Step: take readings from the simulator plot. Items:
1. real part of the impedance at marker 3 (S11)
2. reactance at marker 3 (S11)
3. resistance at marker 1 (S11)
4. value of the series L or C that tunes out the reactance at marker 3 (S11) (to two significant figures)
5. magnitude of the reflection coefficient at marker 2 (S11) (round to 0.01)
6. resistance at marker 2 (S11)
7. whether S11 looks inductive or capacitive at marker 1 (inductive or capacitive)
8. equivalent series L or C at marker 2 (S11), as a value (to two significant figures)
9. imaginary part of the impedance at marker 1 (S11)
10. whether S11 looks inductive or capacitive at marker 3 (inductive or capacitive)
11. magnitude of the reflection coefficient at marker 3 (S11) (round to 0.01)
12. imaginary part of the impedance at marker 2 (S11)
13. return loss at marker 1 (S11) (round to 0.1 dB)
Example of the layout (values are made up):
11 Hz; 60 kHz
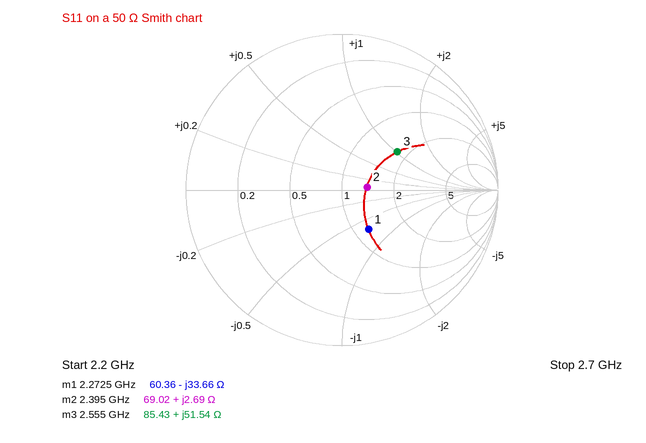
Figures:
85.43 Ω; +51.54 Ω; 60.36 Ω; 1.2 pF; 0.16; 69.02 Ω; capacitive; 180 pH; -33.66 Ω; inductive; 0.43; +2.69 Ω; 10.3 dB
